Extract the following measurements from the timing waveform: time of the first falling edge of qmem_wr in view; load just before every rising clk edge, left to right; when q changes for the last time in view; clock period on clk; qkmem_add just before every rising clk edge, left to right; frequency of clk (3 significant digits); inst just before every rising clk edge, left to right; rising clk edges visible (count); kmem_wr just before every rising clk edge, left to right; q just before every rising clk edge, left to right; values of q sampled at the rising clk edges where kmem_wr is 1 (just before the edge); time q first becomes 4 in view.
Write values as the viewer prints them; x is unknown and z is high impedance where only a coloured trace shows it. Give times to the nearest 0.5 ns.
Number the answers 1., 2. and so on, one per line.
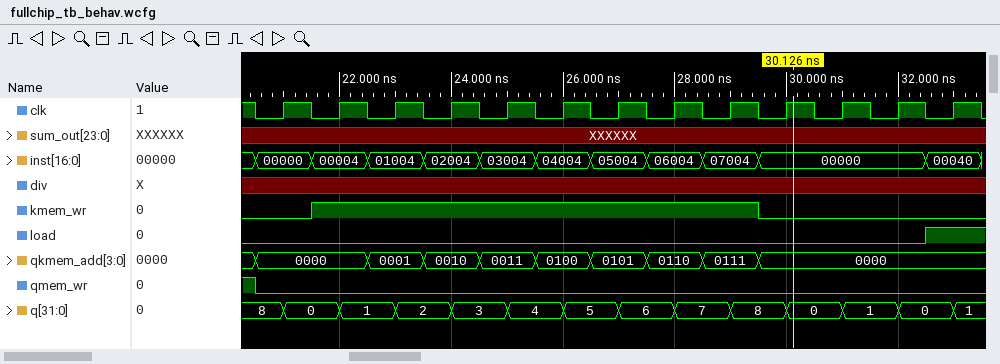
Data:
1. 20.5 ns
2. 0 0 0 0 0 0 0 0 0 0 0 0 1
3. 33 ns
4. 1 ns
5. 0000, 0000, 0001, 0010, 0011, 0100, 0101, 0110, 0111, 0000, 0000, 0000, 0000
6. 1.00 GHz
7. 00000, 00004, 01004, 02004, 03004, 04004, 05004, 06004, 07004, 00000, 00000, 00000, 00040
8. 13
9. 0 1 1 1 1 1 1 1 1 0 0 0 0
10. 8, 0, 1, 2, 3, 4, 5, 6, 7, 8, 0, 1, 0
11. 0, 1, 2, 3, 4, 5, 6, 7
12. 25 ns
